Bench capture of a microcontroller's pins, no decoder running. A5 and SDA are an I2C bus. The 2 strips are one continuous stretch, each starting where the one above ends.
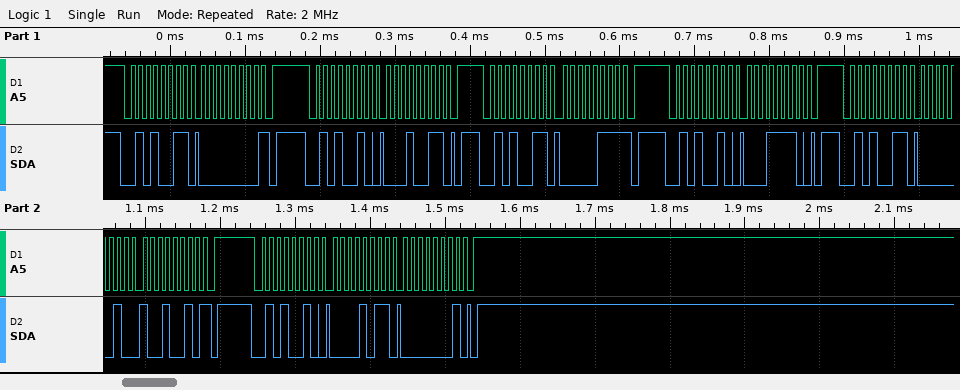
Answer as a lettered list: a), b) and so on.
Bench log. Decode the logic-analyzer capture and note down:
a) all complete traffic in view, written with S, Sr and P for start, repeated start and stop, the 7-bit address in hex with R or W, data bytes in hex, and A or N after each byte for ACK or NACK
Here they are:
a) S 29R A 00 N P S 29W A 13 A P S 29R A 07 N P S 29W A 1E A P S 29R A 02 A 92 N P S 29W A 0B A 01 A P
